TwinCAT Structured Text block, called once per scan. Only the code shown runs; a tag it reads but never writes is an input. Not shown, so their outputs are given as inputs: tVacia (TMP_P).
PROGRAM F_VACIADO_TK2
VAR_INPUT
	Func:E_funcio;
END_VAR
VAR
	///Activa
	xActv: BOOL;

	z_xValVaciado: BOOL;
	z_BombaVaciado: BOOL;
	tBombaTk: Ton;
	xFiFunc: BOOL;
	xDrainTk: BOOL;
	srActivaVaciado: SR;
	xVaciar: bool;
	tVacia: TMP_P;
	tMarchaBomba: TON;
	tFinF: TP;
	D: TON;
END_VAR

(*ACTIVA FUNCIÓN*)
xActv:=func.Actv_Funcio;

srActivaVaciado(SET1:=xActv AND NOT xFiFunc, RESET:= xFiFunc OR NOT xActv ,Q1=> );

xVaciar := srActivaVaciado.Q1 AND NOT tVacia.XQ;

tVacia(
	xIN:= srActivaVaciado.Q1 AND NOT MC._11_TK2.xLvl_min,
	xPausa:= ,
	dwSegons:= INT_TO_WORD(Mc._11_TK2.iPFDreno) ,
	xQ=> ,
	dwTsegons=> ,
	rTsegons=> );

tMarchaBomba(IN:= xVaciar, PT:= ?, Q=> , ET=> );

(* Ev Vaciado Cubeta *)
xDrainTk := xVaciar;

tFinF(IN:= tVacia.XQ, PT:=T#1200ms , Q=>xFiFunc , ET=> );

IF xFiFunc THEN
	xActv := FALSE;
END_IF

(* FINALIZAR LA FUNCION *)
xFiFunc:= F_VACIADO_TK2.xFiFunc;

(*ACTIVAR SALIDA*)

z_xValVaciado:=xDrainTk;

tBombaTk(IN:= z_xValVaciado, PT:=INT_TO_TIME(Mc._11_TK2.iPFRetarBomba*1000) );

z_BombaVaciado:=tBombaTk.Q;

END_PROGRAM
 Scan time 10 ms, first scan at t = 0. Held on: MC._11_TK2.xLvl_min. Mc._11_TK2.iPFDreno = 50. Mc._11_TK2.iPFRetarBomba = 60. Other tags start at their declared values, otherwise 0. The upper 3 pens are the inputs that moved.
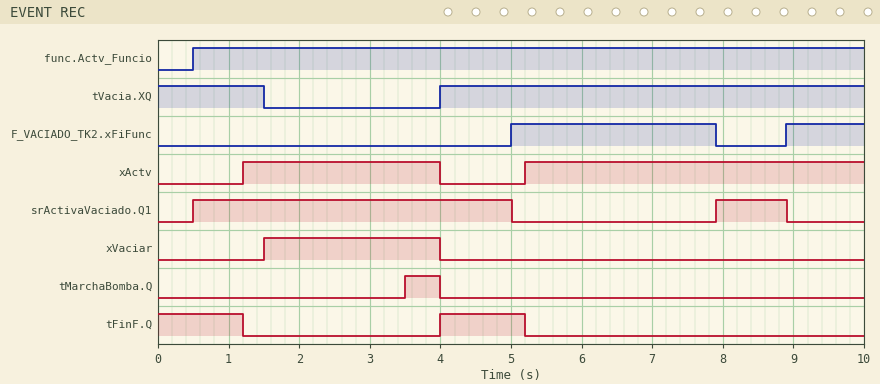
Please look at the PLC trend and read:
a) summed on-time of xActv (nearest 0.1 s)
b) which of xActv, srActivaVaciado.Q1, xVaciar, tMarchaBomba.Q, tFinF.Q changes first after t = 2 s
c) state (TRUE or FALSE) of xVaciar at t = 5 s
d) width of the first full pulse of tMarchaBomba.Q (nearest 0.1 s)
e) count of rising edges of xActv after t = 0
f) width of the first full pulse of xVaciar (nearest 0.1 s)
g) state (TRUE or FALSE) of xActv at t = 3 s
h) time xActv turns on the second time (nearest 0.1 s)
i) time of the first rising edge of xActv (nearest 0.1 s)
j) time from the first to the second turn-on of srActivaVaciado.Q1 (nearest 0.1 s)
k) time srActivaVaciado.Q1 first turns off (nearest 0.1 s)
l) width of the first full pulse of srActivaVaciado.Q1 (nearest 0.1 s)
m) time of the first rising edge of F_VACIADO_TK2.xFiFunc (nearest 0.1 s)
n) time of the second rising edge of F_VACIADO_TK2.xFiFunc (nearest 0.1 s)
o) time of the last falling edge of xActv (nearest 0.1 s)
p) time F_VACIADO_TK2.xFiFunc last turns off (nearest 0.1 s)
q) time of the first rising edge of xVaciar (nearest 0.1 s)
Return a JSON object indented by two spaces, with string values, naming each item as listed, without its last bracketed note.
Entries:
{
  "summed on-time of xActv": "7.6 s",
  "which of xActv, srActivaVaciado.Q1, xVaciar, tMarchaBomba.Q, tFinF.Q changes first after t = 2 s": "tMarchaBomba.Q",
  "state (TRUE or FALSE) of xVaciar at t = 5 s": "FALSE",
  "width of the first full pulse of tMarchaBomba.Q": "0.5 s",
  "count of rising edges of xActv after t = 0": "2",
  "width of the first full pulse of xVaciar": "2.5 s",
  "state (TRUE or FALSE) of xActv at t = 3 s": "TRUE",
  "time xActv turns on the second time": "5.2 s",
  "time of the first rising edge of xActv": "1.2 s",
  "time from the first to the second turn-on of srActivaVaciado.Q1": "7.4 s",
  "time srActivaVaciado.Q1 first turns off": "5.0 s",
  "width of the first full pulse of srActivaVaciado.Q1": "4.5 s",
  "time of the first rising edge of F_VACIADO_TK2.xFiFunc": "5.0 s",
  "time of the second rising edge of F_VACIADO_TK2.xFiFunc": "8.9 s",
  "time of the last falling edge of xActv": "4.0 s",
  "time F_VACIADO_TK2.xFiFunc last turns off": "7.9 s",
  "time of the first rising edge of xVaciar": "1.5 s"
}
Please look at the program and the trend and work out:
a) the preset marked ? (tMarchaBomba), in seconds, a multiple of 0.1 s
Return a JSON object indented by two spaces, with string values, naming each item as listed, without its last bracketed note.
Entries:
{
  "the preset marked ? (tMarchaBomba), in seconds, a multiple of 0.1 s": "2.0 s"
}
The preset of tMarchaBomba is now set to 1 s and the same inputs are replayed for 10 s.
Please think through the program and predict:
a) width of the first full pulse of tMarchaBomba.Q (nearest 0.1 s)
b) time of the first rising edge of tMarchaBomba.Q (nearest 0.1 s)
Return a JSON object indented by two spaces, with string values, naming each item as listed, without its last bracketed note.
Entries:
{
  "width of the first full pulse of tMarchaBomba.Q": "1.5 s",
  "time of the first rising edge of tMarchaBomba.Q": "2.5 s"
}
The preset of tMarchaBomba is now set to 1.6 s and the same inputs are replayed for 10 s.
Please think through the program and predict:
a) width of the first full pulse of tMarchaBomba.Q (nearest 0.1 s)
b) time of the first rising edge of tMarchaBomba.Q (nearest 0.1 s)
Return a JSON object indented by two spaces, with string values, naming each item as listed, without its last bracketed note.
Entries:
{
  "width of the first full pulse of tMarchaBomba.Q": "0.9 s",
  "time of the first rising edge of tMarchaBomba.Q": "3.1 s"
}
